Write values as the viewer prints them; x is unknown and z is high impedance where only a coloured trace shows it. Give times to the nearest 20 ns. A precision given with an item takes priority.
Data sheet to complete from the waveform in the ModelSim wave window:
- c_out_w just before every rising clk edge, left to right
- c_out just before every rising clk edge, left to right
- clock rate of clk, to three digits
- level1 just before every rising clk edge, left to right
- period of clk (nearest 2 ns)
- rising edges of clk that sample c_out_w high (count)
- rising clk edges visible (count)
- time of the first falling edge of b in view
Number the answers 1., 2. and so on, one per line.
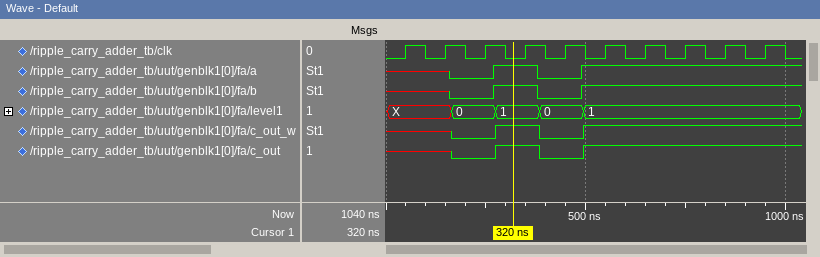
1. x x 0 1 0 1 1 1 1 1
2. x x 0 1 0 1 1 1 1 1
3. 10.0 MHz
4. X, X, 0, 1, 0, 1, 1, 1, 1, 1
5. 100 ns
6. 6
7. 10
8. 380 ns
